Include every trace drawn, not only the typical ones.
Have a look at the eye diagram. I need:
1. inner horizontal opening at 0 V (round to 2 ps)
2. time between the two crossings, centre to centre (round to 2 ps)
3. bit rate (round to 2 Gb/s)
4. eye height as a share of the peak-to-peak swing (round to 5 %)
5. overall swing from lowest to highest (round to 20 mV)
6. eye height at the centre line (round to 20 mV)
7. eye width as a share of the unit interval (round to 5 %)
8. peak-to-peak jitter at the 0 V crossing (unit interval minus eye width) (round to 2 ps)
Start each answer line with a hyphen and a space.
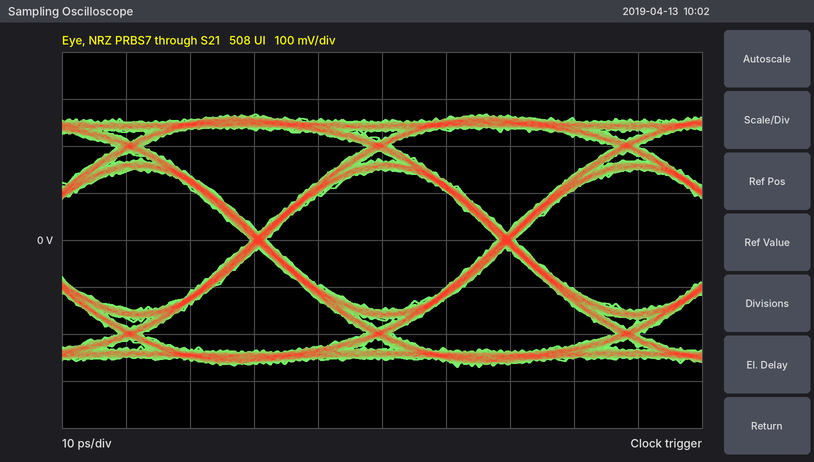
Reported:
- 36 ps
- 38 ps
- 26 Gb/s
- 55 %
- 540 mV
- 300 mV
- 95 %
- 2 ps
